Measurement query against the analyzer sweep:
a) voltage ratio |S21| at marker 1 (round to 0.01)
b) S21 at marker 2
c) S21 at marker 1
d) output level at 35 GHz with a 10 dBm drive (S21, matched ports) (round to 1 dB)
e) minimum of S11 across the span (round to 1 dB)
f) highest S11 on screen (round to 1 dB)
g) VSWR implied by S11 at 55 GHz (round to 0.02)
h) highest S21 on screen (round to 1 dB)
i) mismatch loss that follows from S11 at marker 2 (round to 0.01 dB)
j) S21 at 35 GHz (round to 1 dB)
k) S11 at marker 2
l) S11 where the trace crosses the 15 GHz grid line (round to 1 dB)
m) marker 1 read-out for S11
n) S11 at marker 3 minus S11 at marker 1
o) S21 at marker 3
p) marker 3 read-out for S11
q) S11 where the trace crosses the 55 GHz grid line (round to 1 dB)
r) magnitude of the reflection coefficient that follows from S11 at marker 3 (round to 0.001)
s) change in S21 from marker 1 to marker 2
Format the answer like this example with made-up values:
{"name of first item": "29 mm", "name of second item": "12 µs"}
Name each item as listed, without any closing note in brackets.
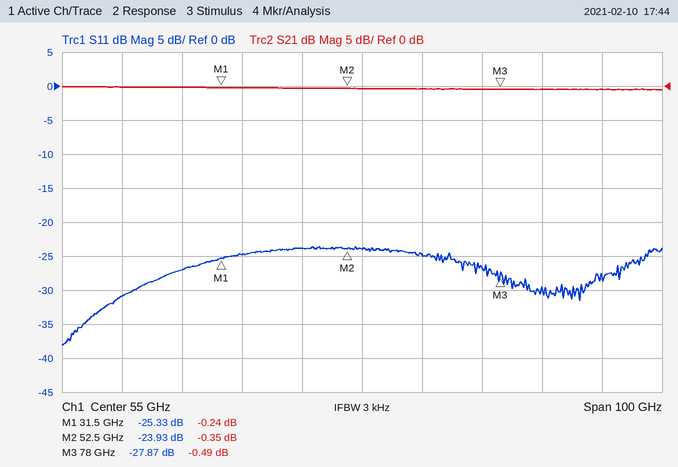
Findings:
{"voltage ratio |S21| at marker 1": "0.97", "S21 at marker 2": "-0.35 dB", "S21 at marker 1": "-0.24 dB", "output level at 35 GHz with a 10 dBm drive (S21, matched ports)": "10 dBm", "minimum of S11 across the span": "-38 dB", "highest S11 on screen": "-24 dB", "VSWR implied by S11 at 55 GHz": "1.14", "highest S21 on screen": "0 dB", "mismatch loss that follows from S11 at marker 2": "0.02 dB", "S21 at 35 GHz": "0 dB", "S11 at marker 2": "-23.93 dB", "S11 where the trace crosses the 15 GHz grid line": "-31 dB", "marker 1 read-out for S11": "-25.33 dB", "S11 at marker 3 minus S11 at marker 1": "-2.54 dB", "S21 at marker 3": "-0.49 dB", "marker 3 read-out for S11": "-27.87 dB", "S11 where the trace crosses the 55 GHz grid line": "-24 dB", "magnitude of the reflection coefficient that follows from S11 at marker 3": "0.040", "change in S21 from marker 1 to marker 2": "-0.11 dB"}
